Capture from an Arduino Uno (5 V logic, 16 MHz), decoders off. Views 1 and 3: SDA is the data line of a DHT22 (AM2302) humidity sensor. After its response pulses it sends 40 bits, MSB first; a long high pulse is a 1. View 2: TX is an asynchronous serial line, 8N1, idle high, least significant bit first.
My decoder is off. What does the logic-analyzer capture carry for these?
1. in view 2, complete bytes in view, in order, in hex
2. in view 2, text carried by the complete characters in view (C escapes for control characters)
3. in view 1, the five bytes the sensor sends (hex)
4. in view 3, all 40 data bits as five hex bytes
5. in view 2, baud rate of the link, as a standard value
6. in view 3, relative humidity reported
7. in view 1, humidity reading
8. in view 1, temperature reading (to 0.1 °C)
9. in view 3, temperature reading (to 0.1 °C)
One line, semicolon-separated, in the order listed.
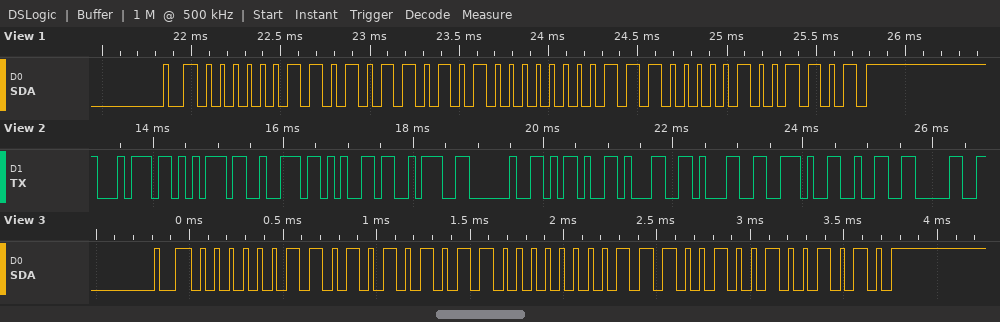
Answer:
74 75 72 65 3A 20 2D 31 31 2E 32 30; "ture: -11.20"; 03 5A 80 70 4D; 03 55 80 72 4A; 9600 baud; 85.3 %; 85.8 %; -11.2 °C; -11.4 °C
